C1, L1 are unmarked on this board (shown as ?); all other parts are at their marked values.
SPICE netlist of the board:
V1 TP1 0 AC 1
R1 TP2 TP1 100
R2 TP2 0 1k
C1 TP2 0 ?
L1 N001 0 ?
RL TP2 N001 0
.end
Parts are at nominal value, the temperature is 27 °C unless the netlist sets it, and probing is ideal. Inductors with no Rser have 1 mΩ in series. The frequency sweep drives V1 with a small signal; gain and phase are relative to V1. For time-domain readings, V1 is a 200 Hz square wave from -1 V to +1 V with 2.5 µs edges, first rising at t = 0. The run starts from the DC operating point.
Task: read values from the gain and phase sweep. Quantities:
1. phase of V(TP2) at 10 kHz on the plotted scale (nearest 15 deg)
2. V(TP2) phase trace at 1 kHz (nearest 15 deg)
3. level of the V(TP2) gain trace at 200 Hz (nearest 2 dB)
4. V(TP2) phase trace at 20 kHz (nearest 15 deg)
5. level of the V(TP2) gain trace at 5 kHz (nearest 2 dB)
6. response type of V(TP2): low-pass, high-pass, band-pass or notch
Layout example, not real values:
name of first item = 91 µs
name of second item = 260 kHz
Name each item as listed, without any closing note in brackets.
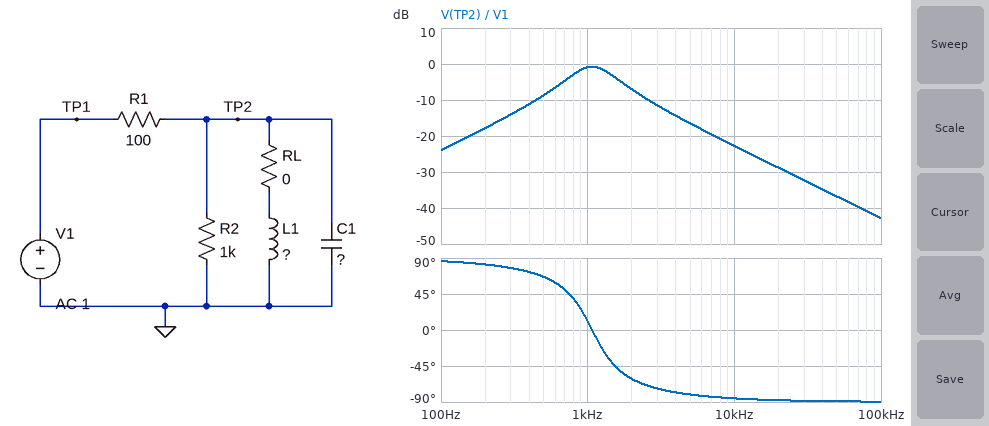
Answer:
phase of V(TP2) at 10 kHz on the plotted scale = -90 deg
V(TP2) phase trace at 1 kHz = 15 deg
level of the V(TP2) gain trace at 200 Hz = -18 dB
V(TP2) phase trace at 20 kHz = -90 deg
level of the V(TP2) gain trace at 5 kHz = -16 dB
response type of V(TP2): low-pass, high-pass, band-pass or notch = band-pass
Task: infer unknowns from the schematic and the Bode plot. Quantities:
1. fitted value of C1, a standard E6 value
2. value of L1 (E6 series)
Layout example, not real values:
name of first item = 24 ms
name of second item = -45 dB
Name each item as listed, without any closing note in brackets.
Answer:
fitted value of C1, a standard E6 value = 2.2 µF
value of L1 = 10 mH
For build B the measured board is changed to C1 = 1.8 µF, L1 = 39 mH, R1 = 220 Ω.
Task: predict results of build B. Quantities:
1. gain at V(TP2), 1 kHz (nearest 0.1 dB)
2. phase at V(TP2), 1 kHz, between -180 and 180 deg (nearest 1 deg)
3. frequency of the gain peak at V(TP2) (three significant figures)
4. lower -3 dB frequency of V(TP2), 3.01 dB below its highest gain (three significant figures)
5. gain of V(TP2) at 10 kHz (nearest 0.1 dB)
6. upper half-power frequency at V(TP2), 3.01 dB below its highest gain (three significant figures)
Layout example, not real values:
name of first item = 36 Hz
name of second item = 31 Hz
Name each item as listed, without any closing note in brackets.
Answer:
gain at V(TP2), 1 kHz = -6.0 dB
phase at V(TP2), 1 kHz, between -180 and 180 deg = -53 deg
frequency of the gain peak at V(TP2) = 601 Hz
lower -3 dB frequency of V(TP2), 3.01 dB below its highest gain = 405 Hz
gain of V(TP2) at 10 kHz = -27.9 dB
upper half-power frequency at V(TP2), 3.01 dB below its highest gain = 891 Hz
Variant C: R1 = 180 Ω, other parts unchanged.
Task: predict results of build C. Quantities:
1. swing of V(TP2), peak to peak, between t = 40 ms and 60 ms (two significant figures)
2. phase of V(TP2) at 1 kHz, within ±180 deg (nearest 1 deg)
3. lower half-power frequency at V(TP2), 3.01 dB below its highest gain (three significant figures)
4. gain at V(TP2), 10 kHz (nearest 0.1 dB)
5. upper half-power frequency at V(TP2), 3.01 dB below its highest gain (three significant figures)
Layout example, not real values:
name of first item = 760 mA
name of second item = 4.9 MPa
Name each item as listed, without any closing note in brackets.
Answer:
swing of V(TP2), peak to peak, between t = 40 ms and 60 ms = 1.1 V
phase of V(TP2) at 1 kHz, within ±180 deg = 17 deg
lower half-power frequency at V(TP2), 3.01 dB below its highest gain = 857 Hz
gain at V(TP2), 10 kHz = -27.8 dB
upper half-power frequency at V(TP2), 3.01 dB below its highest gain = 1.34 kHz
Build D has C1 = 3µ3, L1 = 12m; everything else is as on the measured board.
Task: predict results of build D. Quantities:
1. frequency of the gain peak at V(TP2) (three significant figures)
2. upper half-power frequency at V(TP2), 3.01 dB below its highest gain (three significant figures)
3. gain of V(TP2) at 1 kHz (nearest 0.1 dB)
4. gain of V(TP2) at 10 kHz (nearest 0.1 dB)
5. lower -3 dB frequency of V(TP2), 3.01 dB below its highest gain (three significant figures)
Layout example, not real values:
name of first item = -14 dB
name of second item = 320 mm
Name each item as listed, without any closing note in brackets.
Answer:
frequency of the gain peak at V(TP2) = 800 Hz
upper half-power frequency at V(TP2), 3.01 dB below its highest gain = 1.10 kHz
gain of V(TP2) at 1 kHz = -2.4 dB
gain of V(TP2) at 10 kHz = -26.3 dB
lower -3 dB frequency of V(TP2), 3.01 dB below its highest gain = 580 Hz
